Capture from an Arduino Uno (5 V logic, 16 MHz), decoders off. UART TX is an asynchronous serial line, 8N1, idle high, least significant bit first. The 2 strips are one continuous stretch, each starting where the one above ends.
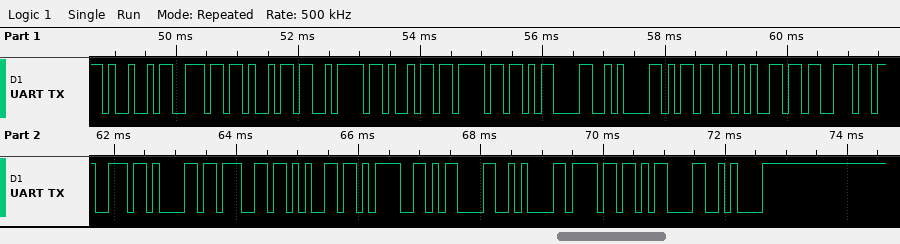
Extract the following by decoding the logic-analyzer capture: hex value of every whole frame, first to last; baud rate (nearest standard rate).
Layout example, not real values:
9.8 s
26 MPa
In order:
0x49 0x6E 0x69 0x7A 0x69 0x6F 0x0D 0x0A 0x6D 0x65 0x73 0x73 0x61 0x67 0x65 0x3D 0x0D 0x0A 0x6F 0x0D 0x0A
9600 baud
